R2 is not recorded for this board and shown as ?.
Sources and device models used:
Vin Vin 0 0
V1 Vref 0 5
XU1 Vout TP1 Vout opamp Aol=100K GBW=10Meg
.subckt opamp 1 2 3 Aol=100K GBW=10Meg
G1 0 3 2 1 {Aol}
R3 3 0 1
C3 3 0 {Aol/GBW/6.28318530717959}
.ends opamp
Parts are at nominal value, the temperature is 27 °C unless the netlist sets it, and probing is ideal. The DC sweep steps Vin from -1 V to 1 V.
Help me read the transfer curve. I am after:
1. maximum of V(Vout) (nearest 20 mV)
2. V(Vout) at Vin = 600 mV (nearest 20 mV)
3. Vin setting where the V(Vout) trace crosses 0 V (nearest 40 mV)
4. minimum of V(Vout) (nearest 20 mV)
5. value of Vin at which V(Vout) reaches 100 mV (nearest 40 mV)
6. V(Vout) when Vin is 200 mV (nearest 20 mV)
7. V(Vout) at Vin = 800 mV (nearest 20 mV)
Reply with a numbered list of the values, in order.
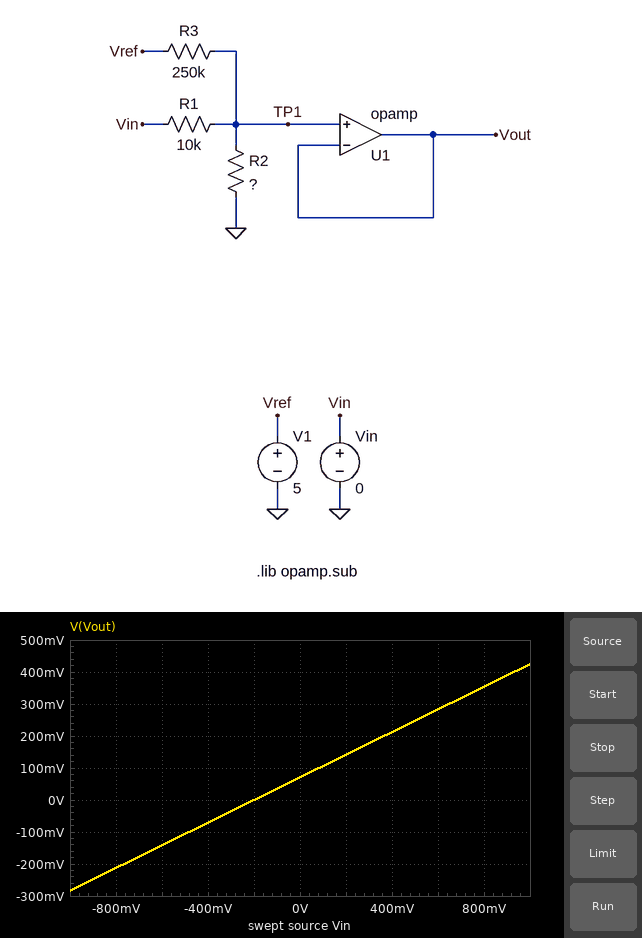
1. 420 mV
2. 280 mV
3. -200 mV
4. -280 mV
5. 80 mV
6. 140 mV
7. 360 mV
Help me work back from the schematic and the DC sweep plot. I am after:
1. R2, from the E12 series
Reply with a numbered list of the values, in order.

1. 5.6 kΩ
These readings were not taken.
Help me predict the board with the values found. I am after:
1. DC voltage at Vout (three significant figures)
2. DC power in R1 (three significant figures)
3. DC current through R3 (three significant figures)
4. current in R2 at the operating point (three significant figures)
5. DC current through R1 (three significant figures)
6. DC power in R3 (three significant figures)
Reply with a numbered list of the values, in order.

1. 70.8 mV
2. 501 nW
3. 19.7 µA
4. 12.6 µA
5. 7.08 µA
6. 97.2 µW
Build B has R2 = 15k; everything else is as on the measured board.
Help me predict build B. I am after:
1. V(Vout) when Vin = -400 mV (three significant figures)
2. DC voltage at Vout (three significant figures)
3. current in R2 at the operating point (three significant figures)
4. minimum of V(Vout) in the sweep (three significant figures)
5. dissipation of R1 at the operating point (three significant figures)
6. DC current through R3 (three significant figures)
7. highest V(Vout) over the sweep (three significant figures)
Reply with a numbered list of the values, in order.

1. -117 mV
2. 117 mV
3. 7.81 µA
4. -469 mV
5. 1.37 µW
6. 19.5 µA
7. 703 mV
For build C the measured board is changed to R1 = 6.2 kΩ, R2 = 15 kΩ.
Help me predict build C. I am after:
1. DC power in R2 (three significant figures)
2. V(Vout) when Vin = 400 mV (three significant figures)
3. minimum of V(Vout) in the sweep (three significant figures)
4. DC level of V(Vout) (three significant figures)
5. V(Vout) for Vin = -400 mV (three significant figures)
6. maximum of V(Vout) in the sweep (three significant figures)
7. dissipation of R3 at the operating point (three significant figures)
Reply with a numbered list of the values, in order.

1. 496 nW
2. 364 mV
3. -609 mV
4. 86.2 mV
5. -192 mV
6. 782 mV
7. 96.6 µW
